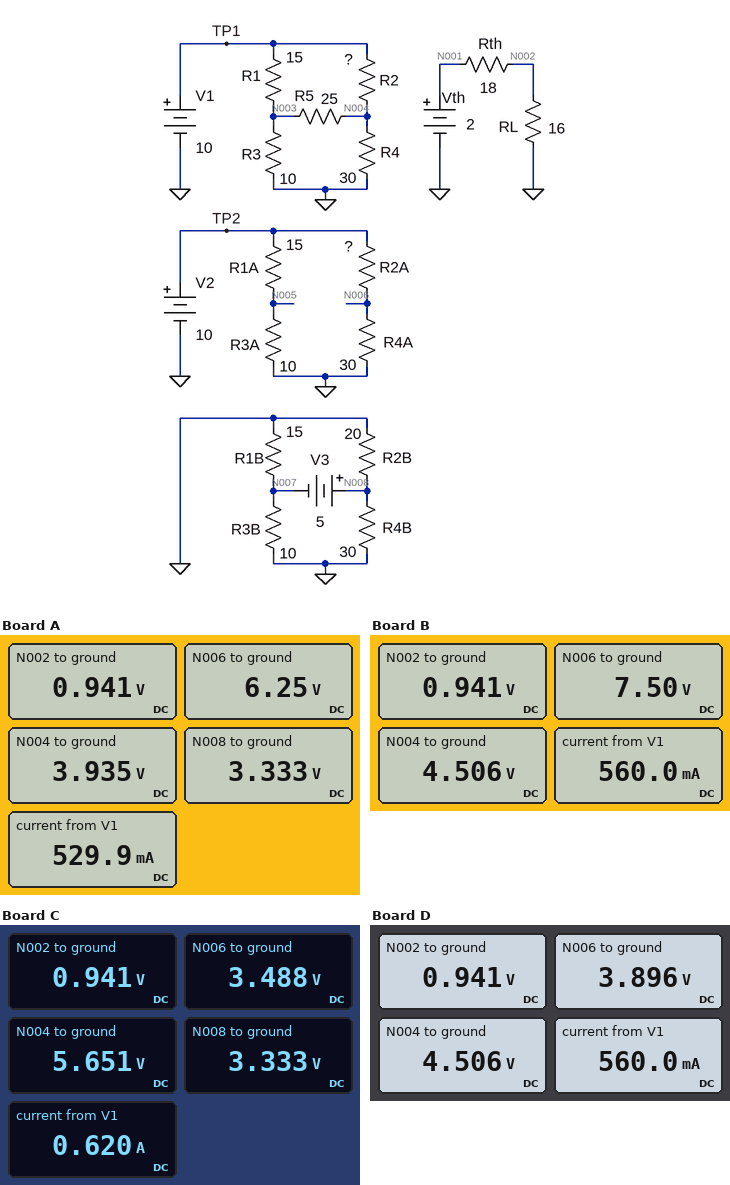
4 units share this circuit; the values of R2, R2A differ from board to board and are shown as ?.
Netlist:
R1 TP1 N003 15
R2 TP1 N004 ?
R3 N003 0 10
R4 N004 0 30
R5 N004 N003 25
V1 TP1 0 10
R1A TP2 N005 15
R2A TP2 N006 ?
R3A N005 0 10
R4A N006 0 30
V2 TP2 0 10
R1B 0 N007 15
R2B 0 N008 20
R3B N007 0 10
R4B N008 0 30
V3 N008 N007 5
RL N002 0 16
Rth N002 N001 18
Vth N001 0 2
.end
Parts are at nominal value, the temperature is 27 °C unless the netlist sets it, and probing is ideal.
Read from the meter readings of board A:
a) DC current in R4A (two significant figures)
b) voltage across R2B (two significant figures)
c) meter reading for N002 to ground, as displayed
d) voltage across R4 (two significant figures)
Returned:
210 mA
3.3 V
0.941 V
3.9 V
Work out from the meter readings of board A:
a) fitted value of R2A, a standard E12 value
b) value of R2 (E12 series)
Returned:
18 Ω
47 Ω
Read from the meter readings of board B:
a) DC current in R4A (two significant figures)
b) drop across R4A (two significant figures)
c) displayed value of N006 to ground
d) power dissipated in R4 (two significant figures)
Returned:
250 mA
7.5 V
7.50 V
680 mW
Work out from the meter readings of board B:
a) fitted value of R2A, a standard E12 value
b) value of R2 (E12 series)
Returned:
10 Ω
33 Ω
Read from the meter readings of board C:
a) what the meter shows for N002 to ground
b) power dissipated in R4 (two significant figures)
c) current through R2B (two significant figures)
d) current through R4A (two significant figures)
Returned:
0.941 V
1.1 W
170 mA
120 mA
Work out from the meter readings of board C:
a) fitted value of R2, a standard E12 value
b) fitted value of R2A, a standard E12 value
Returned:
18 Ω
56 Ω
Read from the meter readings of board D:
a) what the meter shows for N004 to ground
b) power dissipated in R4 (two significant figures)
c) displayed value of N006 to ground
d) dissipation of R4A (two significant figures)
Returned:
4.506 V
680 mW
3.896 V
510 mW
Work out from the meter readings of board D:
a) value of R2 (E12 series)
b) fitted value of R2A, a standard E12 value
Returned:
33 Ω
47 Ω
